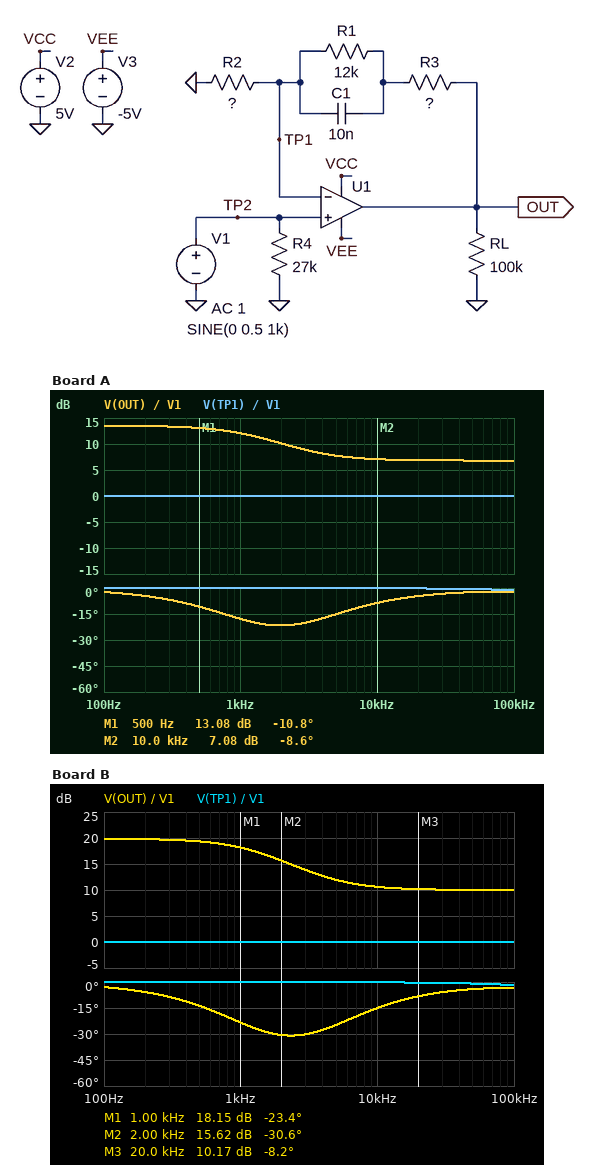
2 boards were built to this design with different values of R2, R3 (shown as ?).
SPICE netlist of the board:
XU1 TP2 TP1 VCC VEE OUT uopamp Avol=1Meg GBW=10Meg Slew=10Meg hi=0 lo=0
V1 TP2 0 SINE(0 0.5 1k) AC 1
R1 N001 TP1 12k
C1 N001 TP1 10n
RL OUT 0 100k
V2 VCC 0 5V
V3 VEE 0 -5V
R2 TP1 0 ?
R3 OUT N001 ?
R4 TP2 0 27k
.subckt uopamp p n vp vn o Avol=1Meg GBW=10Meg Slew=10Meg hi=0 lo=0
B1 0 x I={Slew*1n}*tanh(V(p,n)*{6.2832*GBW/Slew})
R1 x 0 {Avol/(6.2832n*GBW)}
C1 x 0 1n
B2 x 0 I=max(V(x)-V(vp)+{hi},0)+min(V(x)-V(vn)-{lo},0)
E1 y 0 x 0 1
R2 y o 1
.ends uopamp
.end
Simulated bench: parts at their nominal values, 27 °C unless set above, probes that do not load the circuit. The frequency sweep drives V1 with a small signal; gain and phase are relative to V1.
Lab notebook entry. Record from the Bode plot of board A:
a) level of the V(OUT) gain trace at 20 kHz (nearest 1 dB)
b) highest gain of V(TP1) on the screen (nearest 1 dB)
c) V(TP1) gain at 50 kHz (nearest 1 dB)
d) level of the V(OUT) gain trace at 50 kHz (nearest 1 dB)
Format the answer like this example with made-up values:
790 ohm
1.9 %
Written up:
7 dB
0 dB
0 dB
7 dB
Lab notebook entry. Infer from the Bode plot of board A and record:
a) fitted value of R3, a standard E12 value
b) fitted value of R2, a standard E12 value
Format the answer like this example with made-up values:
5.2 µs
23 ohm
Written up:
5.6 kΩ
4.7 kΩ
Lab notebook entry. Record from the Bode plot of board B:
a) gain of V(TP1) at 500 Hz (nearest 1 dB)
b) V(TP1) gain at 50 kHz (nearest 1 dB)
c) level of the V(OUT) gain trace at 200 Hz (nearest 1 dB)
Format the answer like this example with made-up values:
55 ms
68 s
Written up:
0 dB
0 dB
20 dB
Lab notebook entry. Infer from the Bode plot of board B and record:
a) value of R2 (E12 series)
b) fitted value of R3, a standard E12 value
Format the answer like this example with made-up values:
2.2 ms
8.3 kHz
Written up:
1.8 kΩ
3.9 kΩ
